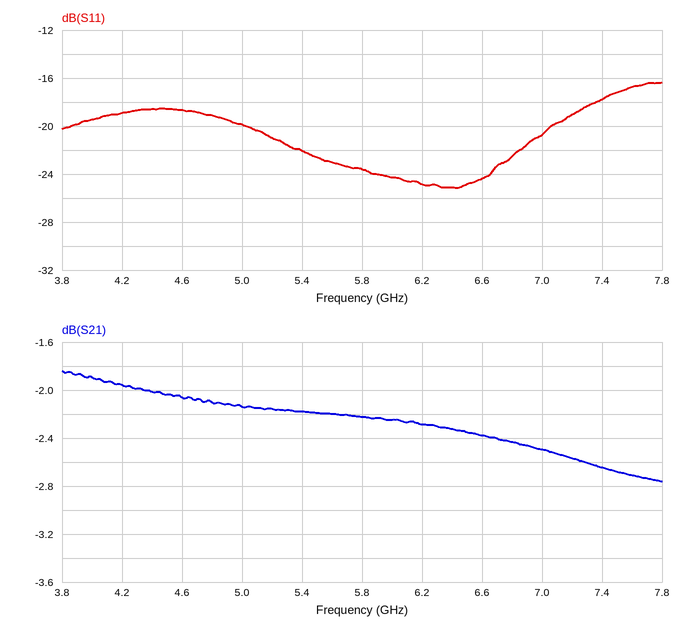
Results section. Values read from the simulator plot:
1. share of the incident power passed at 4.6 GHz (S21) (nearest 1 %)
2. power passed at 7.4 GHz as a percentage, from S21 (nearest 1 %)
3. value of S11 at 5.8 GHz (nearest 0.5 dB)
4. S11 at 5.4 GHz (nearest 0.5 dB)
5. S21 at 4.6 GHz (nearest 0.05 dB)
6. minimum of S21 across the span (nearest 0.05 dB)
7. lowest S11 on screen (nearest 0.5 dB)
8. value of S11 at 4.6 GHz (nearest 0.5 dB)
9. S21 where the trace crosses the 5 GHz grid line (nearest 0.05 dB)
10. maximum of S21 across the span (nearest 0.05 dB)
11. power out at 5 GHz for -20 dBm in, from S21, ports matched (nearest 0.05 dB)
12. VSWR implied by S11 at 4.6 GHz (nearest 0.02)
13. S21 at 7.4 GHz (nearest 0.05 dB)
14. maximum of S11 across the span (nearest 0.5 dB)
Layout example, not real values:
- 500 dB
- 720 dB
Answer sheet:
- 62 %
- 54 %
- -23.5 dB
- -22.0 dB
- -2.05 dB
- -2.75 dB
- -25.0 dB
- -18.5 dB
- -2.15 dB
- -1.85 dB
- -22.15 dBm
- 1.26
- -2.65 dB
- -16.5 dB
